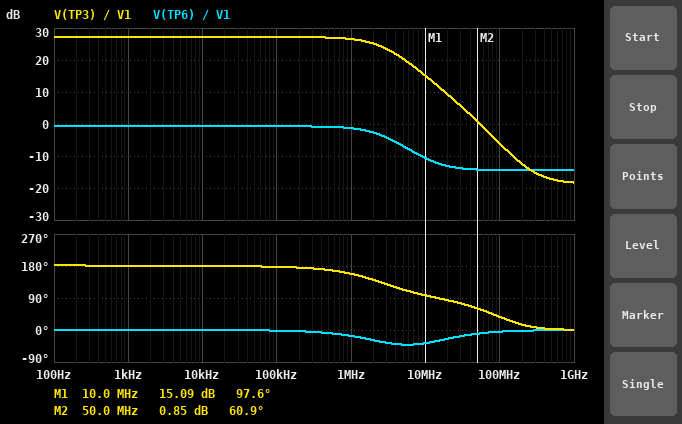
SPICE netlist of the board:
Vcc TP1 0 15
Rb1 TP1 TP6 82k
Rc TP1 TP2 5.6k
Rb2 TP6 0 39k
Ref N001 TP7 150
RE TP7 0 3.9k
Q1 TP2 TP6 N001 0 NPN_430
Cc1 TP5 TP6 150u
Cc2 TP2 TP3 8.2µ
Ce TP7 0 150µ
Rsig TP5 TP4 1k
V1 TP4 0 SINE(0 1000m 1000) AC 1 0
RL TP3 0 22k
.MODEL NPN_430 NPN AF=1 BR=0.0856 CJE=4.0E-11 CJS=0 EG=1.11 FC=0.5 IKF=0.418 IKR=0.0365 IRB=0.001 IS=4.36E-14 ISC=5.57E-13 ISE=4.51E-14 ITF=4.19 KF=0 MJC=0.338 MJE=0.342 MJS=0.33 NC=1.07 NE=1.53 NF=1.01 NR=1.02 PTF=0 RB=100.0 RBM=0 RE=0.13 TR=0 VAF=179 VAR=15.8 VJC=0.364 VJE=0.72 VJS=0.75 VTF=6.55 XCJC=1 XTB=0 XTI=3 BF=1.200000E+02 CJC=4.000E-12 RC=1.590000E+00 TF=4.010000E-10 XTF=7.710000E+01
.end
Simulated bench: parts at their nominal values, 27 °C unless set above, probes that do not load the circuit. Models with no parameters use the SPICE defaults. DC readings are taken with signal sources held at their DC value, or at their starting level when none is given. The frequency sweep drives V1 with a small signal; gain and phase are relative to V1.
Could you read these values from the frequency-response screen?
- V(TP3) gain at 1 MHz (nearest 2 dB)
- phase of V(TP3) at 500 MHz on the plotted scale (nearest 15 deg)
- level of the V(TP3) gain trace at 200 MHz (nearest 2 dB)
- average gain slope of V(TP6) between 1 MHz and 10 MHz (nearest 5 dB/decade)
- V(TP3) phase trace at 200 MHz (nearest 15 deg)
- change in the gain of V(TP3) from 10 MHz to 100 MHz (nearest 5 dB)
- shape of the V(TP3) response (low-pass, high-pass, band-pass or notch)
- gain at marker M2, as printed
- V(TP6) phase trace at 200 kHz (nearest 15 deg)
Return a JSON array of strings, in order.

["26 dB", "0 deg", "-12 dB", "-10 dB/decade", "15 deg", "-20 dB", "low-pass", "0.85 dB", "0 deg"]
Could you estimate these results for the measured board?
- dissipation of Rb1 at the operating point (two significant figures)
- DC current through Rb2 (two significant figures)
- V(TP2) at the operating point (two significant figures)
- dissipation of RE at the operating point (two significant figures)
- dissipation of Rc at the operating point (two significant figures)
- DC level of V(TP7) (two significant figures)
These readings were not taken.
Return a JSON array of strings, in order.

["1.3 mW", "120 µA", "9.5 V", "3.8 mW", "5.3 mW", "3.8 V"]
